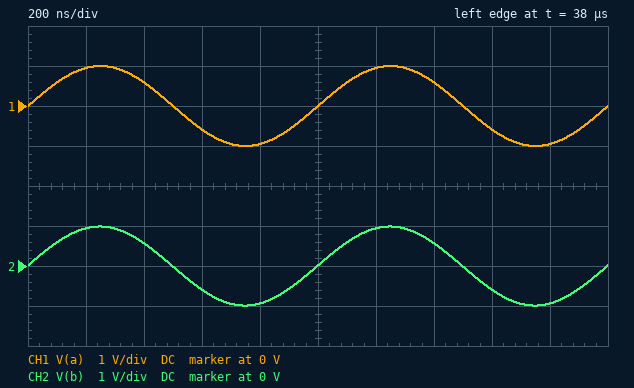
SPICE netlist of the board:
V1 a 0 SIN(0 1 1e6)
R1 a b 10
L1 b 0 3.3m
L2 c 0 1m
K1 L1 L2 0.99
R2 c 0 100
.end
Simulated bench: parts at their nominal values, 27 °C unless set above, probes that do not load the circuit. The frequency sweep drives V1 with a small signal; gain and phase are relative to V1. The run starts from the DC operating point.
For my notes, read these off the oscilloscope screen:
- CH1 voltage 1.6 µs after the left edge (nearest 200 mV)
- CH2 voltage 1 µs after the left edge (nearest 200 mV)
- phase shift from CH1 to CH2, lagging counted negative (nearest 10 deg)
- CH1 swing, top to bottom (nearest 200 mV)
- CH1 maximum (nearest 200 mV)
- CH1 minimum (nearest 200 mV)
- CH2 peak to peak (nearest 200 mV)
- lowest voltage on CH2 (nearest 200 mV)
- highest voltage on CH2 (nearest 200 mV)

-600 mV
0 V
0 deg
2.0 V
1.0 V
-1.0 V
2.0 V
-1.0 V
1.0 V
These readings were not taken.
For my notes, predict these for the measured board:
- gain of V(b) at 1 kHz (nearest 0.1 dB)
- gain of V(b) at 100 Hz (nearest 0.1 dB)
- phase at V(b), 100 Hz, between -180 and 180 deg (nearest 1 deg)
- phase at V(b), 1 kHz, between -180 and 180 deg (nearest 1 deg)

-1.1 dB
-13.9 dB
78 deg
25 deg
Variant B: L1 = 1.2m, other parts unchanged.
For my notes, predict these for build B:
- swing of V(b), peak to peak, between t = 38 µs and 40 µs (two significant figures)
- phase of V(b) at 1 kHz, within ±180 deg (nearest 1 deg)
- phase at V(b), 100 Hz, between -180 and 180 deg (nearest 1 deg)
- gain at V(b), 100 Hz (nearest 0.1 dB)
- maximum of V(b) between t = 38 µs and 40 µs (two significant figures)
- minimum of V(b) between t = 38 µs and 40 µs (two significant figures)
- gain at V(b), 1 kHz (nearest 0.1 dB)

1.9 V
51 deg
85 deg
-22.5 dB
970 mV
-970 mV
-4.7 dB
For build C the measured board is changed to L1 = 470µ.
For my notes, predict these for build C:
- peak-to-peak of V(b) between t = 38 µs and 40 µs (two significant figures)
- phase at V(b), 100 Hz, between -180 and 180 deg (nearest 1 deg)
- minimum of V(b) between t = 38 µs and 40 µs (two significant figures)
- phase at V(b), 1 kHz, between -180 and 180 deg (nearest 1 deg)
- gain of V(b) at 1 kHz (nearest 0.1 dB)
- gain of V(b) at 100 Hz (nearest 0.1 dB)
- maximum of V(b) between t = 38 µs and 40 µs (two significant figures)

1.8 V
88 deg
-920 mV
70 deg
-11.1 dB
-30.6 dB
920 mV
